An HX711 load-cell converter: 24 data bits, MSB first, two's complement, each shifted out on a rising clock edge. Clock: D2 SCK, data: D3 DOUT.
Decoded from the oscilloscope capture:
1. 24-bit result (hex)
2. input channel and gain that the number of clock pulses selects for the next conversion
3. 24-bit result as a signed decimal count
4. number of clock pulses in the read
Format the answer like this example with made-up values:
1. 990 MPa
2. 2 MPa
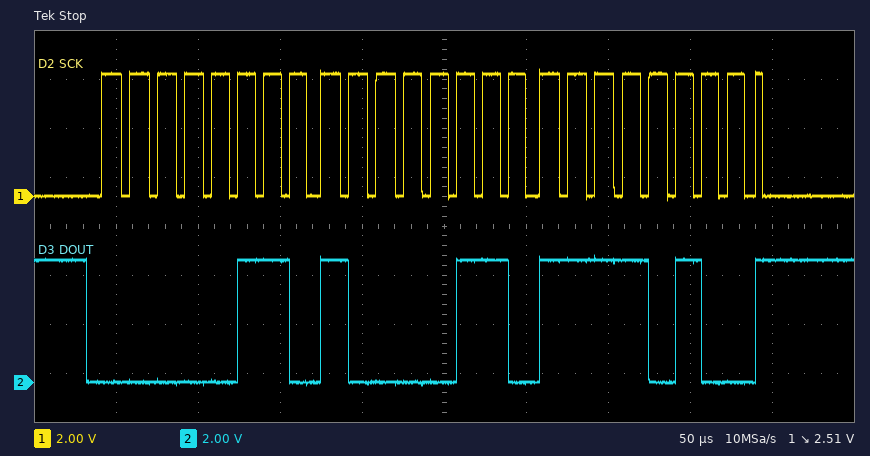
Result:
1. 0x0686F4
2. channel A, gain 128
3. 427764
4. 25
